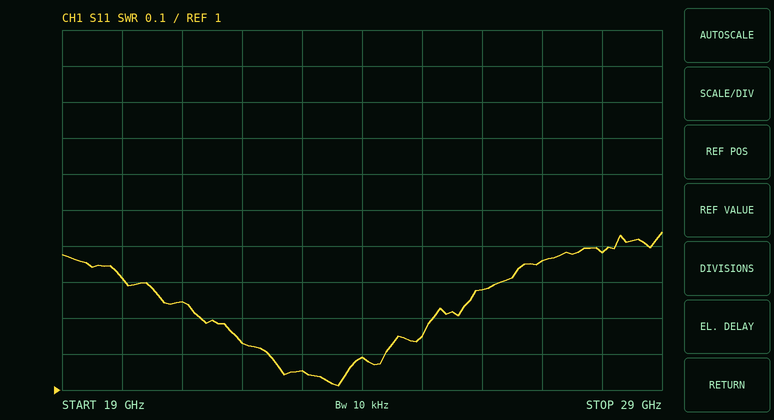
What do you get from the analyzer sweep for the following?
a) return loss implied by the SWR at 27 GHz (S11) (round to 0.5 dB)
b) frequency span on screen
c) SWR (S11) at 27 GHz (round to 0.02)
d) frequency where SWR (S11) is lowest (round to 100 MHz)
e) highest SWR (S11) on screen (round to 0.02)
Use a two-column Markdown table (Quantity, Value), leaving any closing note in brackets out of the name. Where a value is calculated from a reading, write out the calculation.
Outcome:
| Quantity | Value |
|---|---|
| return loss implied by the SWR at 27 GHz (S11) | −20 log10((1.36 − 1)/(1.36 + 1)) ≈ 16.3 dB, so 16.5 dB to the nearest 0.5 dB |
| frequency span on screen | 10 GHz |
| SWR (S11) at 27 GHz | 1.36 |
| frequency where SWR (S11) is lowest | 23.6 GHz |
| highest SWR (S11) on screen | 1.44 |
